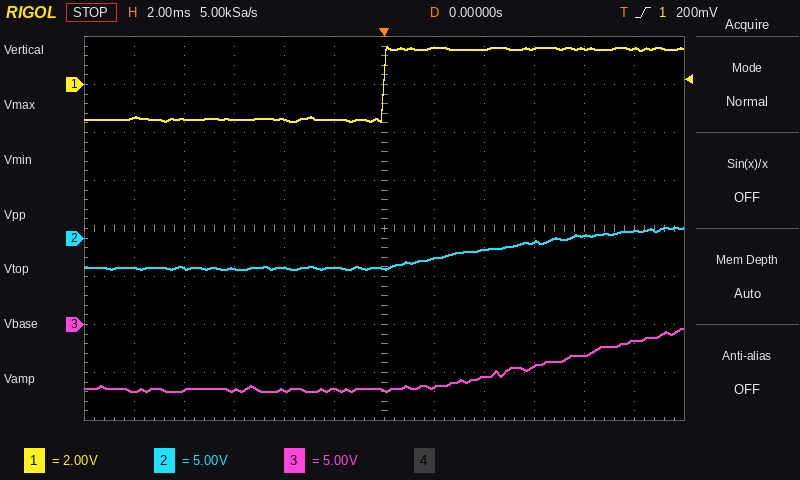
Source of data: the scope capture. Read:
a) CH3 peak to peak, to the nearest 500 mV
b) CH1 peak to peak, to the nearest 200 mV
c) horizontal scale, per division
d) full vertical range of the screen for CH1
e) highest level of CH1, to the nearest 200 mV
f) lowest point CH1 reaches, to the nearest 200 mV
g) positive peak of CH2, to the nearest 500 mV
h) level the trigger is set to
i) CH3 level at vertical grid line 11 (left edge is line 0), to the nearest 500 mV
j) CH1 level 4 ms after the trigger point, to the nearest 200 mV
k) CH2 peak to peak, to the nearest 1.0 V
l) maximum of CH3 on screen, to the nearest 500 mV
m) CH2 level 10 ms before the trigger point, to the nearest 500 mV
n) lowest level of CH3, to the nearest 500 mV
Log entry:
6.5 V
3.2 V
2 ms
16 V
1.6 V
-1.6 V
1.0 V
200 mV
-1.5 V
1.4 V
4.0 V
-500 mV
-3.0 V
-7.0 V
